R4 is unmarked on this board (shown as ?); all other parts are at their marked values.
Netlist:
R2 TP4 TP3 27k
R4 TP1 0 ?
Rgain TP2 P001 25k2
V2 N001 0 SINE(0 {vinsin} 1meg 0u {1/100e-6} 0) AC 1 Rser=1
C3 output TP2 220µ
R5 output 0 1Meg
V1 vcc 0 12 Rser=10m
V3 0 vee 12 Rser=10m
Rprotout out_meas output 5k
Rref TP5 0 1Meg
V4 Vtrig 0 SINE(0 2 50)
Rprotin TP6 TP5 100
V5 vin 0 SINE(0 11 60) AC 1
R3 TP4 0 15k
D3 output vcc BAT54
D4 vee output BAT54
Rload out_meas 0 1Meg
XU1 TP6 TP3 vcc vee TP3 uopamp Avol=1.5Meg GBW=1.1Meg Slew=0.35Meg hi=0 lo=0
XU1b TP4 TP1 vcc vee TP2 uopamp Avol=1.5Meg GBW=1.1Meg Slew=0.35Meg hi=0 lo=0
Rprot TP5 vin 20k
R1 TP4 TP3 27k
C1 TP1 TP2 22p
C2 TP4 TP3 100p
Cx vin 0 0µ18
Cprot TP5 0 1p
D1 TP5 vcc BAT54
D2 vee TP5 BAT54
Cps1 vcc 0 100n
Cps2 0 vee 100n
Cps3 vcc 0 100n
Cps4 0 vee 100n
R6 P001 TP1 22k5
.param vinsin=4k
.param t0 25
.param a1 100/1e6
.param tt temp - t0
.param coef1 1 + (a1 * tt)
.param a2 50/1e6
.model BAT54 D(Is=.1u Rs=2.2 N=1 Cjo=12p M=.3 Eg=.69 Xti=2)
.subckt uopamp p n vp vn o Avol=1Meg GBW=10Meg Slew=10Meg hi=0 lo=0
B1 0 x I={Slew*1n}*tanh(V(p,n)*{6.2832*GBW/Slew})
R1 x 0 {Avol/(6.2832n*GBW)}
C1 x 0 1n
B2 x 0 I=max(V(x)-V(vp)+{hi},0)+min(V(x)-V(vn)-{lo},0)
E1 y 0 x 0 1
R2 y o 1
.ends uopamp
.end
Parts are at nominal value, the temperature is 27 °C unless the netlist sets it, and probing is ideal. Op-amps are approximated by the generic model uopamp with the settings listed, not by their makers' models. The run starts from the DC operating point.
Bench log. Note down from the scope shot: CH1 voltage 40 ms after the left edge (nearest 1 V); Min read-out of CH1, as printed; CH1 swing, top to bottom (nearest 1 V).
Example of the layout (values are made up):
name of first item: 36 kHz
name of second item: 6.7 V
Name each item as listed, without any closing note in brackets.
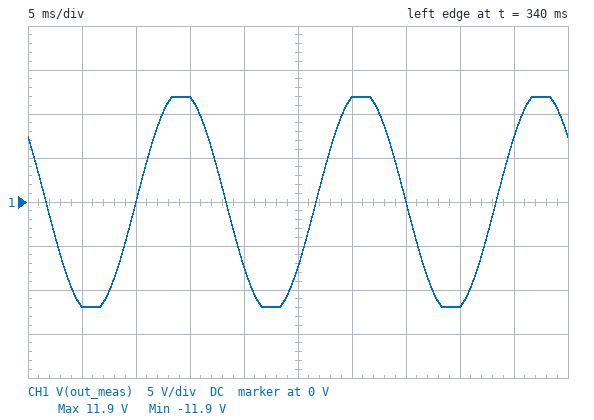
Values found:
CH1 voltage 40 ms after the left edge: -12 V
Min read-out of CH1, as printed: -11.9 V
CH1 swing, top to bottom: 24 V
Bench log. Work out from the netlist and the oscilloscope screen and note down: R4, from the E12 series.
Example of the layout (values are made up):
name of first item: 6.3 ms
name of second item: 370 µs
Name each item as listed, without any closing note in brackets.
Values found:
R4, from the E12 series: 39 kΩ
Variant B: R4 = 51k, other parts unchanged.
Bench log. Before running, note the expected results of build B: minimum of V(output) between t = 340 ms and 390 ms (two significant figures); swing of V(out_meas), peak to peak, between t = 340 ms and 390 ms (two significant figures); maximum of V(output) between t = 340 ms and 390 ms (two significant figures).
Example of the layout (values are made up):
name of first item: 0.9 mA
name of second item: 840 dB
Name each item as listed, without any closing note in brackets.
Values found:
minimum of V(output) between t = 340 ms and 390 ms: -11 V
swing of V(out_meas), peak to peak, between t = 340 ms and 390 ms: 22 V
maximum of V(output) between t = 340 ms and 390 ms: 11 V
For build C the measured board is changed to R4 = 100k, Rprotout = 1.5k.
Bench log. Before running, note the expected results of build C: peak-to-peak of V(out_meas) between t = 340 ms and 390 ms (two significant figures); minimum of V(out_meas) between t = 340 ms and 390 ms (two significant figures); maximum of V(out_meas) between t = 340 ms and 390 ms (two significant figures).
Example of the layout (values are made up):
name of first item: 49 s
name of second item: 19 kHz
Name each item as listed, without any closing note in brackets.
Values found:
peak-to-peak of V(out_meas) between t = 340 ms and 390 ms: 17 V
minimum of V(out_meas) between t = 340 ms and 390 ms: -8.4 V
maximum of V(out_meas) between t = 340 ms and 390 ms: 8.4 V
